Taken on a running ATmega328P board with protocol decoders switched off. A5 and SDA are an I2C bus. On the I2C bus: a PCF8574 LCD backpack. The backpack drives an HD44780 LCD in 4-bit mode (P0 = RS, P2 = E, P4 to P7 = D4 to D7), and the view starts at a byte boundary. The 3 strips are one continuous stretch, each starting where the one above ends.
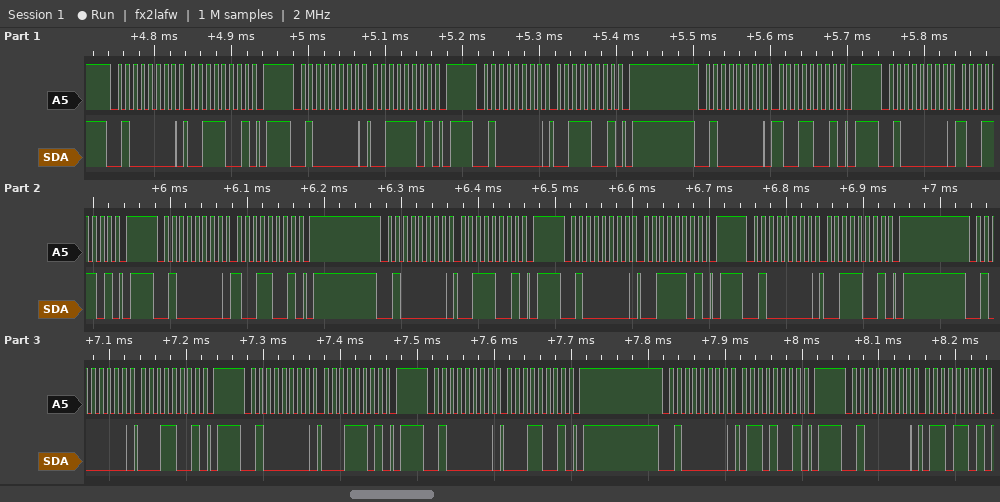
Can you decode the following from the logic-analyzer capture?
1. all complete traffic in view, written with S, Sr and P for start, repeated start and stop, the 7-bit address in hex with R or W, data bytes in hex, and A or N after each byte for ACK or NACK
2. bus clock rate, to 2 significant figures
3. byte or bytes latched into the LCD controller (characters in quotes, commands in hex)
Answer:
S 20W A 39 A P S 20W A 3D A P S 20W A 39 A P S 20W A 99 A P S 20W A 9D A P S 20W A 99 A P S 20W A 39 A P S 20W A 3D A P S 20W A 39 A P S 20W A 19 A P S 20W A 1D A P S 20W A 19 A P S 20W A 69 A P S 20W A 6D A
100 kHz
'9' '1'
